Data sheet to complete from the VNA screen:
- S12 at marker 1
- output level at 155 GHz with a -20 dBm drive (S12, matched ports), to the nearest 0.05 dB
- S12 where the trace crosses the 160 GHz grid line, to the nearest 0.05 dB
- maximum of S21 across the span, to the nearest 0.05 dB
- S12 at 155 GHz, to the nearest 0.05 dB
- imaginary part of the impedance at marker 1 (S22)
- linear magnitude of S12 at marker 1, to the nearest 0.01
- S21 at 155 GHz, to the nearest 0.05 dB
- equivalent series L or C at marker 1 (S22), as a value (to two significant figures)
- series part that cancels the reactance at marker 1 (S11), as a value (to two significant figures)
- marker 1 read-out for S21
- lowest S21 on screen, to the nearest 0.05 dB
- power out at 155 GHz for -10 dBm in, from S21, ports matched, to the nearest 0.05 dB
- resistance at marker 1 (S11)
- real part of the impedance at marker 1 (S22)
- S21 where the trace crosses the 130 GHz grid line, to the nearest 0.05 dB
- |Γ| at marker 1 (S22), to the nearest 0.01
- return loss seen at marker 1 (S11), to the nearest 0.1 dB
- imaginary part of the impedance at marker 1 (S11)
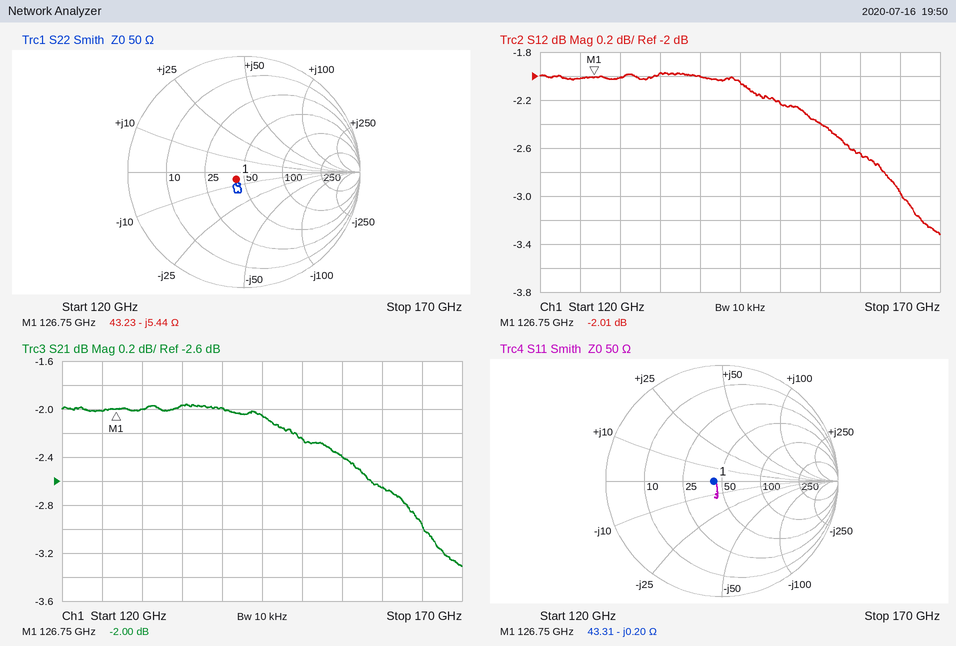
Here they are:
-2.01 dB
-22.40 dBm
-2.65 dB
-1.95 dB
-2.40 dB
-5.44 Ω
0.79
-2.40 dB
230 fF
250 fH
-2.00 dB
-3.30 dB
-12.40 dBm
43.31 Ω
43.23 Ω
-2.00 dB
0.09
22.9 dB
-0.20 Ω
